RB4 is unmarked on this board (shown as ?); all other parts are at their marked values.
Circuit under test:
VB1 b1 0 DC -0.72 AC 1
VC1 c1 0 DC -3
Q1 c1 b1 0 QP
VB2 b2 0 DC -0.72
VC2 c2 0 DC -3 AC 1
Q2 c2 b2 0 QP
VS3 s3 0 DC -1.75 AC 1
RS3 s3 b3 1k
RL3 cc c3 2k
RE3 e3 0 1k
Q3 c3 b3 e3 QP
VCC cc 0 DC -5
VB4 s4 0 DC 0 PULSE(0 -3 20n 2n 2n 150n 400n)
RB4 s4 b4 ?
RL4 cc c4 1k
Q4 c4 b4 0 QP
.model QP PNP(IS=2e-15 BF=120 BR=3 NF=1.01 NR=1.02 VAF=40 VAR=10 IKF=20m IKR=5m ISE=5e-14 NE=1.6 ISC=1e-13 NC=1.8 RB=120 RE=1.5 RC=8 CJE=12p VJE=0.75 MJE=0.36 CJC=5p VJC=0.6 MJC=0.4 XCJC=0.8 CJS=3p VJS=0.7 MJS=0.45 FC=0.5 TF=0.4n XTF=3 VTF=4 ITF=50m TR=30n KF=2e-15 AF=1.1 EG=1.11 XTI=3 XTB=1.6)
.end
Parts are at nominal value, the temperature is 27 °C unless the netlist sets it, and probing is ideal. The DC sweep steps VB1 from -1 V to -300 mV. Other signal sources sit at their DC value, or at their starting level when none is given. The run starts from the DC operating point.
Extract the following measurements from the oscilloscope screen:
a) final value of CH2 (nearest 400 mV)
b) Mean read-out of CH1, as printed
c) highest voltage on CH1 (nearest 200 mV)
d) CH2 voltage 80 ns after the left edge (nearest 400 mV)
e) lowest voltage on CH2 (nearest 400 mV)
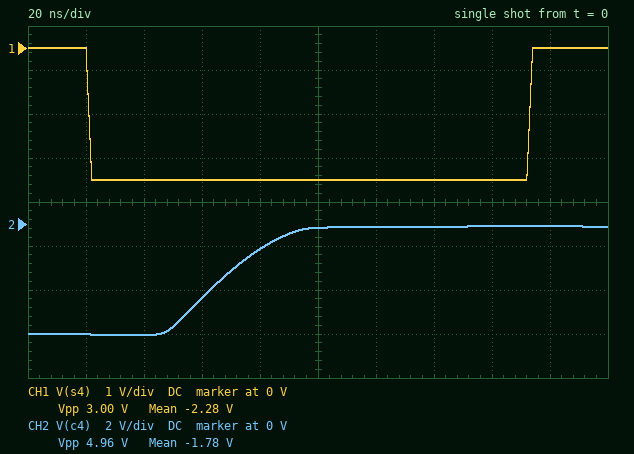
0 V
-2.28 V
0 V
-1.2 V
-5.2 V
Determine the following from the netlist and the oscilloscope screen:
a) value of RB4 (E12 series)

4.7 kΩ
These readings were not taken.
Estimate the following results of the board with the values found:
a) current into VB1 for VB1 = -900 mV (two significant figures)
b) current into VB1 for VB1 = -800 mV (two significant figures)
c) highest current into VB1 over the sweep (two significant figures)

470 µA
120 µA
960 µA
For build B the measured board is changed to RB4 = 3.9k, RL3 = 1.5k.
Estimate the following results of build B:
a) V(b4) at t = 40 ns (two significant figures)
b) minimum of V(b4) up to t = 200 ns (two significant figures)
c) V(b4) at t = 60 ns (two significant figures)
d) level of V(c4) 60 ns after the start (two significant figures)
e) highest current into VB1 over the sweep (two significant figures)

-680 mV
-840 mV
-800 mV
-2.4 V
960 µA
